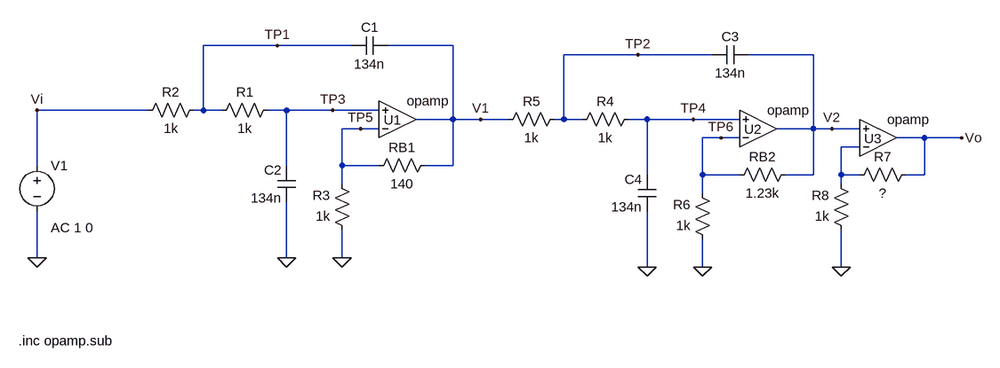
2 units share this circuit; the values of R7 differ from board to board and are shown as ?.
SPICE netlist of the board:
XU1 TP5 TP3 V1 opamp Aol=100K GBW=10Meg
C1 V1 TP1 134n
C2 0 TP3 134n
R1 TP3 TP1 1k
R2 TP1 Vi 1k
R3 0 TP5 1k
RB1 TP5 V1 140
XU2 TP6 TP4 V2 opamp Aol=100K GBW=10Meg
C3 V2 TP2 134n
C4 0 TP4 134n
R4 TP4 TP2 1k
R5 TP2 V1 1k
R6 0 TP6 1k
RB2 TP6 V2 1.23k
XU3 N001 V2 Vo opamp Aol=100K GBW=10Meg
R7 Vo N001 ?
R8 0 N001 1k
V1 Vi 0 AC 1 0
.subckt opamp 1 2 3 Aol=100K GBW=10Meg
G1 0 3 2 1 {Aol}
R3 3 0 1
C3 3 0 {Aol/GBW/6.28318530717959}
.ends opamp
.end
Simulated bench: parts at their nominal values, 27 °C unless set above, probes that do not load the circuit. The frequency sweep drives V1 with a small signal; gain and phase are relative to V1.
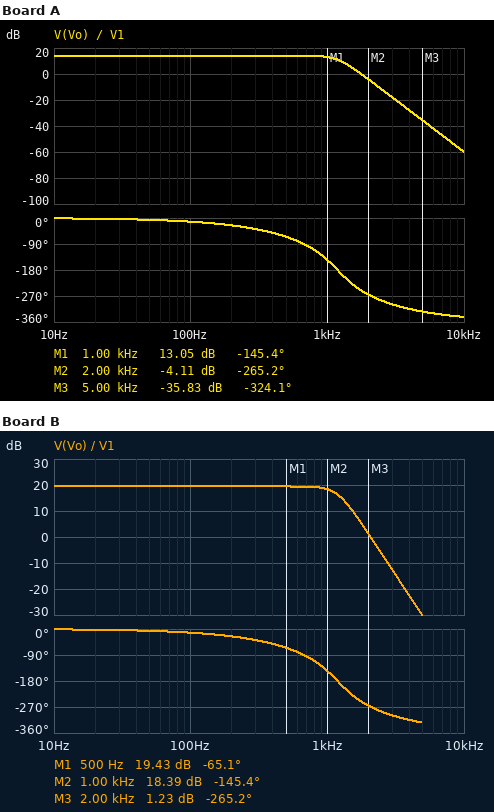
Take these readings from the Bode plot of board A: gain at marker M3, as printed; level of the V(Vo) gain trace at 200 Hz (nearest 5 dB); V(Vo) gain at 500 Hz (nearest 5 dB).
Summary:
-35.83 dB
15 dB
15 dB
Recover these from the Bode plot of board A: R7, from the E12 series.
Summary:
1 kΩ
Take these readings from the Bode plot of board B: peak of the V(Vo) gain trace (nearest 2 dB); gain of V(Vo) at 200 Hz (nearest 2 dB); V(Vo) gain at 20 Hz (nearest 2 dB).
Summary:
20 dB
20 dB
20 dB
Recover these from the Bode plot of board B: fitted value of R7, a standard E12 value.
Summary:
2.7 kΩ
